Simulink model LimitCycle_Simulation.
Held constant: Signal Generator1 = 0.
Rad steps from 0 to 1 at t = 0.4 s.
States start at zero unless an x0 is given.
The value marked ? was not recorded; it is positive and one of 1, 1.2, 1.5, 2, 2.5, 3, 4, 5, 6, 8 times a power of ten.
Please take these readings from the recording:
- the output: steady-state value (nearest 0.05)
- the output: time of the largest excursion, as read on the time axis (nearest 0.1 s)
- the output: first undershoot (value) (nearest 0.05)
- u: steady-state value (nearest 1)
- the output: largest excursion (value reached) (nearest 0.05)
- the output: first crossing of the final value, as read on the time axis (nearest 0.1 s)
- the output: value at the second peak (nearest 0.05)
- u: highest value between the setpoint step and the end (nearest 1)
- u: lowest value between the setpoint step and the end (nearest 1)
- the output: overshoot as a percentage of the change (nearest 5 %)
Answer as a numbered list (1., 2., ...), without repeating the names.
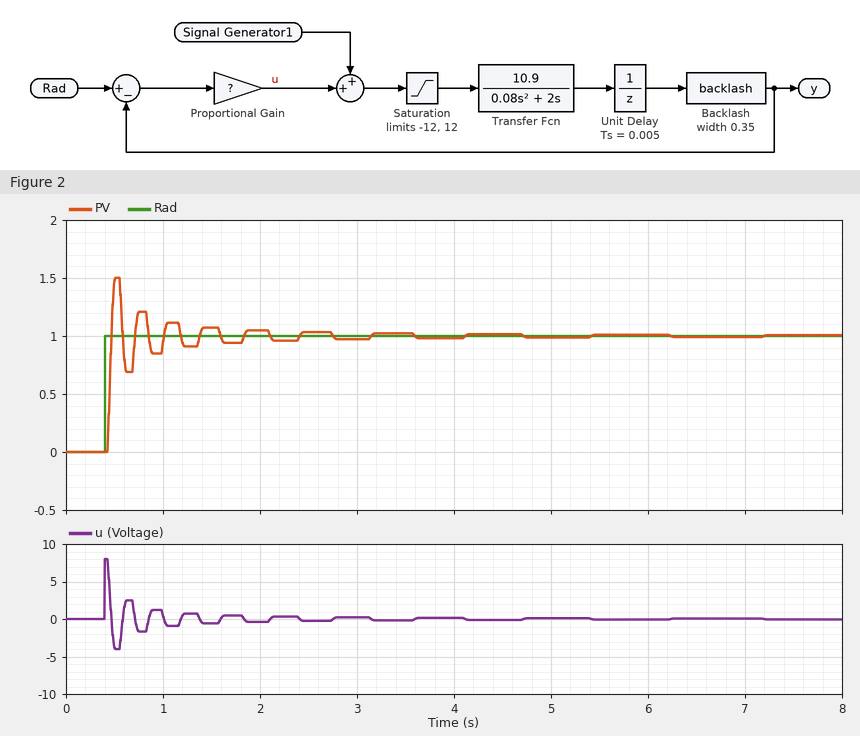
1. 1.00
2. 0.5 s
3. 0.70
4. 0
5. 1.50
6. 0.5 s
7. 1.20
8. 8
9. -4
10. 50 %
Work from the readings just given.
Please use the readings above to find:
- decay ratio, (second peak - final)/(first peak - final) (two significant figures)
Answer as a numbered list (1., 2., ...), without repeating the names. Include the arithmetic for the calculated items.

1. (1.2 - 1) / (1.5 - 1) = 0.40
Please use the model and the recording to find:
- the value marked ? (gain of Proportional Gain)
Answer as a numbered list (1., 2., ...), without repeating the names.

1. 8
